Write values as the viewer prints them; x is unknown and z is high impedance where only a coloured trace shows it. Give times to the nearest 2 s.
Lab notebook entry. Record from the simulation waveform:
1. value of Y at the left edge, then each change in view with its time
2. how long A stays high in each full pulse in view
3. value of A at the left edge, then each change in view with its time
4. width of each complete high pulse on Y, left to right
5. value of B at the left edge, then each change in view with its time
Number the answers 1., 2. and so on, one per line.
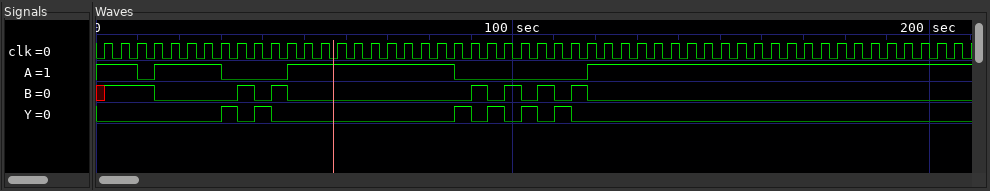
1. 0, 1 at 30 s, 0 at 34 s, 1 at 38 s, 0 at 42 s, 1 at 86 s, 0 at 90 s, 1 at 94 s, 0 at 98 s, 1 at 102 s, 0 at 106 s, 1 at 110 s, 0 at 114 s
2. 16 s, 40 s
3. 1, 0 at 10 s, 1 at 14 s, 0 at 30 s, 1 at 46 s, 0 at 86 s, 1 at 118 s
4. 4 s, 4 s, 4 s, 4 s, 4 s, 4 s
5. x, 1 at 2 s, 0 at 14 s, 1 at 34 s, 0 at 38 s, 1 at 42 s, 0 at 46 s, 1 at 90 s, 0 at 94 s, 1 at 98 s, 0 at 102 s, 1 at 106 s, 0 at 110 s, 1 at 114 s, 0 at 118 s
